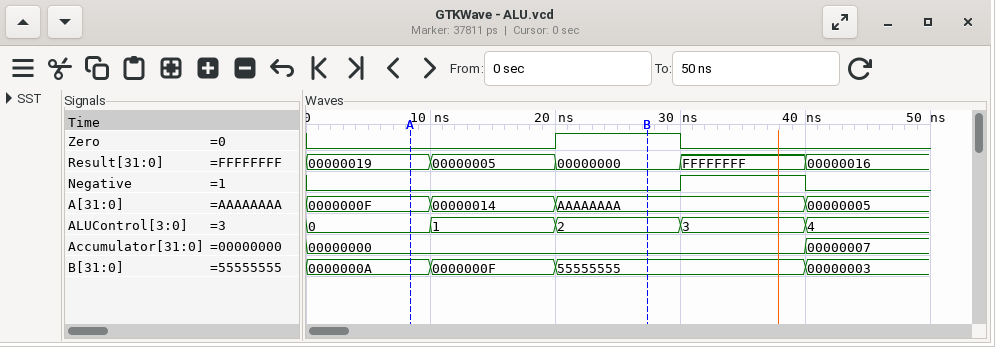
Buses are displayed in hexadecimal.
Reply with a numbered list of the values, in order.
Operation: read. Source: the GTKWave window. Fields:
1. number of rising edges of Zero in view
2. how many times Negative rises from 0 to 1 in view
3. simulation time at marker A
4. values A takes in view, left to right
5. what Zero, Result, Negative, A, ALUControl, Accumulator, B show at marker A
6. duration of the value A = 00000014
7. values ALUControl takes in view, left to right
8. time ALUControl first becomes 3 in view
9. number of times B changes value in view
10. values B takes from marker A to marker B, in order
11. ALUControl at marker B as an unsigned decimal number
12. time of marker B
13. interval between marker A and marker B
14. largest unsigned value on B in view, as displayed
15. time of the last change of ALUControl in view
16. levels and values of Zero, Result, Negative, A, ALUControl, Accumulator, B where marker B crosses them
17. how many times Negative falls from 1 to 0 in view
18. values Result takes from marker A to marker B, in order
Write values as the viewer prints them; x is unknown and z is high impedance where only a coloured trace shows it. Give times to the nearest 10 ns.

1. 1
2. 1
3. 10 ns
4. 0000000F, 00000014, AAAAAAAA, 00000005
5. Zero=0, Result=00000019, Negative=0, A=0000000F, ALUControl=0, Accumulator=00000000, B=0000000A
6. 10 ns
7. 0, 1, 2, 3, 4
8. 30 ns
9. 3
10. 0000000A, 0000000F, 55555555
11. 2
12. 30 ns
13. 20 ns
14. 55555555
15. 40 ns
16. Zero=1, Result=00000000, Negative=0, A=AAAAAAAA, ALUControl=2, Accumulator=00000000, B=55555555
17. 1
18. 00000019, 00000005, 00000000
